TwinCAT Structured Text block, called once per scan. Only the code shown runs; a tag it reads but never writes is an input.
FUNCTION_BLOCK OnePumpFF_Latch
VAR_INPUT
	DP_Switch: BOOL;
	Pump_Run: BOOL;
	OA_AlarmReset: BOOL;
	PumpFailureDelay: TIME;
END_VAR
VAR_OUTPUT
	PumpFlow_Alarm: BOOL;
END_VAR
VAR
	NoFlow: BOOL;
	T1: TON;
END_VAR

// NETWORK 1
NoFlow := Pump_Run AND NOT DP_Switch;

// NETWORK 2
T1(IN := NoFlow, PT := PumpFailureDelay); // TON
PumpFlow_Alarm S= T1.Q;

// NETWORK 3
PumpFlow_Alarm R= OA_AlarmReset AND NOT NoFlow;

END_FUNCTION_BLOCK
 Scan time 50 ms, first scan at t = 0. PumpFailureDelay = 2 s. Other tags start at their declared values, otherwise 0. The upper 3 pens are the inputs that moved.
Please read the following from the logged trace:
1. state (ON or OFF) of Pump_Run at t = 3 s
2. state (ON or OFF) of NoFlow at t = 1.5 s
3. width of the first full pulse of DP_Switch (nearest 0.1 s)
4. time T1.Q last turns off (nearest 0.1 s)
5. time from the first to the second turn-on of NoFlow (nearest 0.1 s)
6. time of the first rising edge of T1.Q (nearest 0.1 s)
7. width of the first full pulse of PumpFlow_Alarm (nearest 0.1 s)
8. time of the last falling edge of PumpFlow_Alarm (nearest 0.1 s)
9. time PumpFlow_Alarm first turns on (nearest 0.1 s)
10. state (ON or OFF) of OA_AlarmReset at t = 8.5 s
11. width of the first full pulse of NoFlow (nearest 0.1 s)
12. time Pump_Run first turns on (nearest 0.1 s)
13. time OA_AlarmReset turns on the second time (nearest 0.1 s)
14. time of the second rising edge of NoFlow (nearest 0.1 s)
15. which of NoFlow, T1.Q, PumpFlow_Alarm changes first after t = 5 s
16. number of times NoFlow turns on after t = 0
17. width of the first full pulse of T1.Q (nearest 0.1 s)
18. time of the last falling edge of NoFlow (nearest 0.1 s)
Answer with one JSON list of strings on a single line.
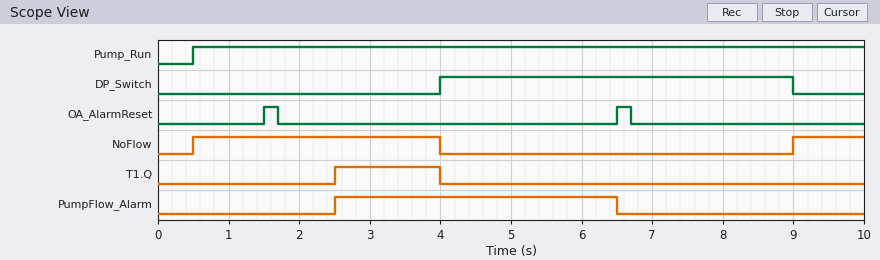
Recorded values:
["ON", "ON", "5.0 s", "4.0 s", "8.5 s", "2.5 s", "4.0 s", "6.5 s", "2.5 s", "OFF", "3.5 s", "0.5 s", "6.5 s", "9.0 s", "PumpFlow_Alarm", "2", "1.5 s", "4.0 s"]
